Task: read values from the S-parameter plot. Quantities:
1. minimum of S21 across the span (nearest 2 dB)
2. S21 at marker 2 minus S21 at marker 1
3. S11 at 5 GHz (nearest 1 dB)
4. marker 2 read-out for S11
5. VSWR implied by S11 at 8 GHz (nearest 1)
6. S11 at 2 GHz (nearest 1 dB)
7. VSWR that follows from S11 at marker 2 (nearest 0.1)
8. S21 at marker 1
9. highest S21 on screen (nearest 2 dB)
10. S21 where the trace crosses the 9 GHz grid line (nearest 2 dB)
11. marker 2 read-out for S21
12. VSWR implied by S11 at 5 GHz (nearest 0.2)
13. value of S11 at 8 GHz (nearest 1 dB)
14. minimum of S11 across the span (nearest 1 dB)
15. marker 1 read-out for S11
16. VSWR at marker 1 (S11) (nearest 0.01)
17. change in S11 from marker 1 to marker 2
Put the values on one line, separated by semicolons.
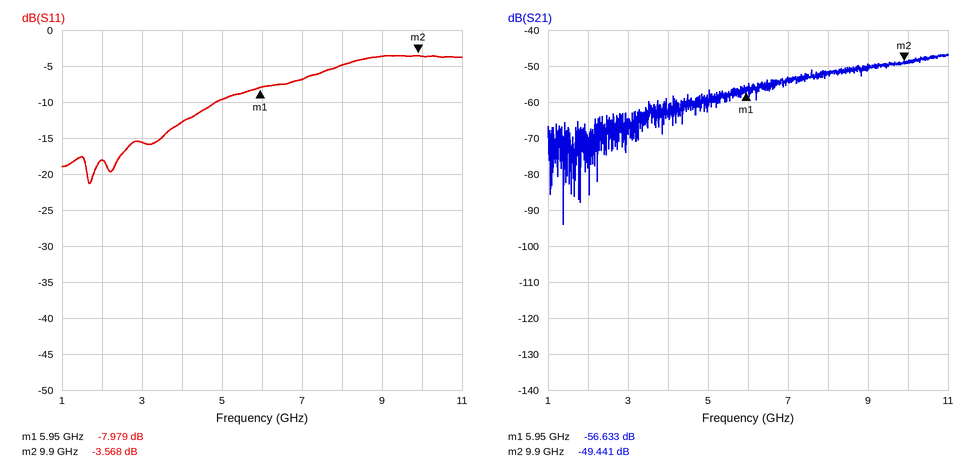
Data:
-94 dB; 7.192 dB; -10 dB; -3.568 dB; 4; -18 dB; 4.9; -56.633 dB; -46 dB; -50 dB; -49.441 dB; 2.0; -5 dB; -21 dB; -7.979 dB; 2.33; 4.411 dB
